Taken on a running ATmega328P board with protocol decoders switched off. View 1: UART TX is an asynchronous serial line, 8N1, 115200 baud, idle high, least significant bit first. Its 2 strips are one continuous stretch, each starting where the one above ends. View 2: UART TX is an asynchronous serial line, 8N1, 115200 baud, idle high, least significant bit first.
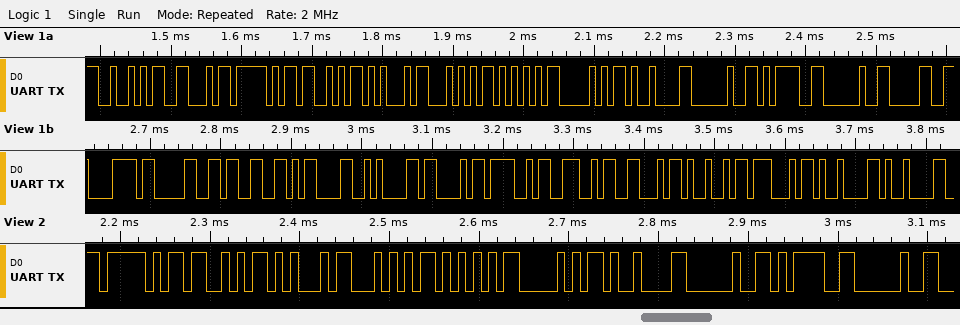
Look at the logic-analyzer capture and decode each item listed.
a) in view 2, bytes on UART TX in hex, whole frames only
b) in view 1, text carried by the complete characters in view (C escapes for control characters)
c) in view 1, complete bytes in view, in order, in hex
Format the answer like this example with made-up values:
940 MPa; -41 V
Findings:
5F 53 45 54 55 50 09 20 3D 20; "RF_SETUP\t = 0x03\r\nCONFIG\t\t"; 52 46 5F 53 45 54 55 50 09 20 3D 20 30 78 30 33 0D 0A 43 4F 4E 46 49 47 09 09
